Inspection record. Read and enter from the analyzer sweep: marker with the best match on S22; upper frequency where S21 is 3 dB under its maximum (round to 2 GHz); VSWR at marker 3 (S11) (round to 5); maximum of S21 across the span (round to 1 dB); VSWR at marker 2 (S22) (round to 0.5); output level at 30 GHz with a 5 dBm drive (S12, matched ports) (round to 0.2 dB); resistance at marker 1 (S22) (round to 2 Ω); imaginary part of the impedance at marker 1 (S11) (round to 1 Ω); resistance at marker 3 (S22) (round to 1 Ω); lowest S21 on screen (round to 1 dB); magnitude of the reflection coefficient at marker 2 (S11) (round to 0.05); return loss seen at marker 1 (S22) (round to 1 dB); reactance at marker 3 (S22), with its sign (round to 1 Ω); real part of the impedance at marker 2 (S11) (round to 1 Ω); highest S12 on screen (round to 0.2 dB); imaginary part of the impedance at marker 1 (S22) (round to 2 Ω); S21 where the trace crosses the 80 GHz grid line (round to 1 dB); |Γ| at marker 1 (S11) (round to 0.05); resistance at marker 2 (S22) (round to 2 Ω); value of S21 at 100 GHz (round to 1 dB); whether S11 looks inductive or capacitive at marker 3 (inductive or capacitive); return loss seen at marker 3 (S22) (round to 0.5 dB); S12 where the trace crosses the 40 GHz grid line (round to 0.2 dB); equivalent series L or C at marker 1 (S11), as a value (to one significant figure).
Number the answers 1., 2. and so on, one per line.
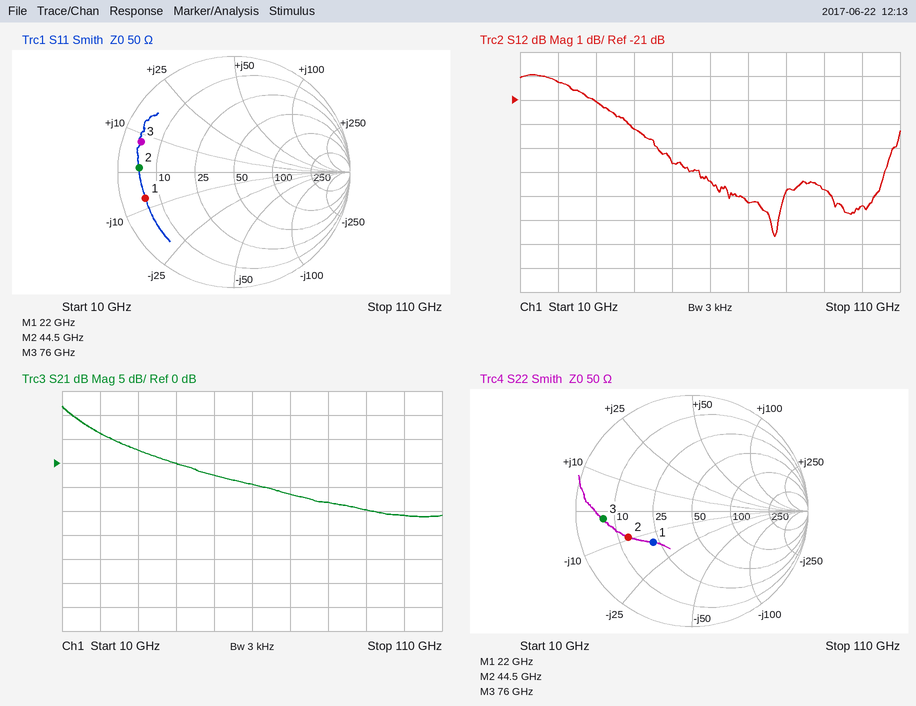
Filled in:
1. marker 1
2. 14 GHz
3. 10
4. 12 dB
5. 4.0
6. -16.0 dBm
7. 22 Ω
8. -7 Ω
9. 7 Ω
10. -11 dB
11. 0.80
12. 7 dB
13. -2 Ω
14. 5 Ω
15. -20.0 dB
16. -14 Ω
17. -8 dB
18. 0.80
19. 14 Ω
20. -11 dB
21. inductive
22. 2.5 dB
23. -22.2 dB
24. 1 pF
